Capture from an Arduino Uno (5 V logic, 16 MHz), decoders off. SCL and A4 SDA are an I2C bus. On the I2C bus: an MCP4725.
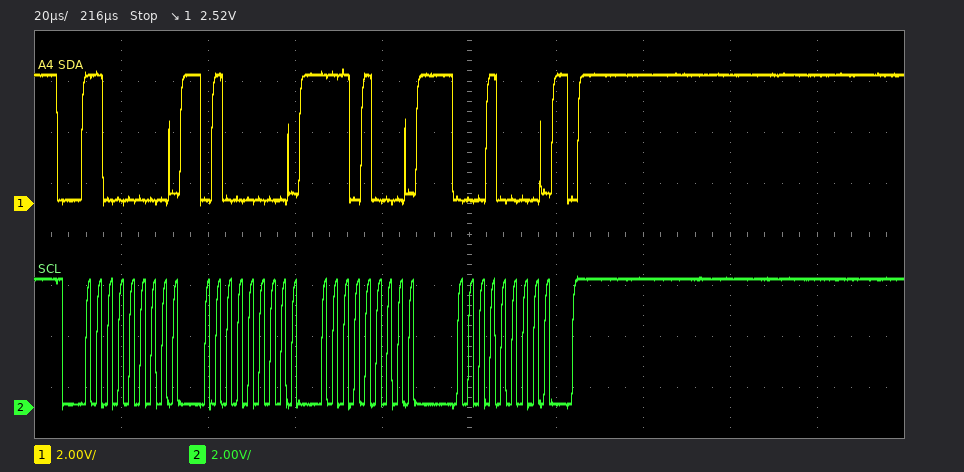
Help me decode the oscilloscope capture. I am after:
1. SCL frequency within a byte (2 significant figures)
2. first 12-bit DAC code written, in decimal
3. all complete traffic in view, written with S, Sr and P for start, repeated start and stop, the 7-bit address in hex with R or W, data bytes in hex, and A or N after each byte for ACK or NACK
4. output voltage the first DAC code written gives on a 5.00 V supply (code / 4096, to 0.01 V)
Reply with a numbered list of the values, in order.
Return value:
1. 400 kHz
2. 3713
3. S 60W A 40 A E8 A 10 A P
4. 4.53 V
